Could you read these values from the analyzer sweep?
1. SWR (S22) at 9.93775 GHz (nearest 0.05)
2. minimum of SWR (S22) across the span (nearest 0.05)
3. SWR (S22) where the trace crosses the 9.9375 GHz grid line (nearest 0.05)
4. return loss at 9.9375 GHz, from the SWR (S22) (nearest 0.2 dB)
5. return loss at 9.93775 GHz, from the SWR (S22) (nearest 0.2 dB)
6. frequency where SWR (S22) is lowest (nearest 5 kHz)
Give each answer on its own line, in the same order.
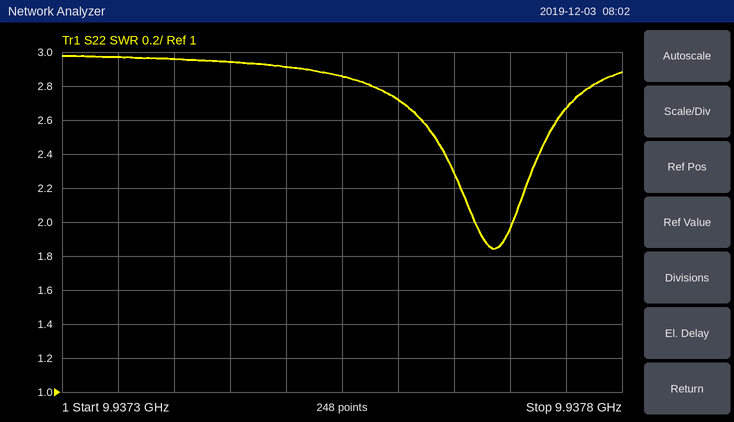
2.65
1.85
2.90
6.2 dB
6.8 dB
9.937685 GHz
